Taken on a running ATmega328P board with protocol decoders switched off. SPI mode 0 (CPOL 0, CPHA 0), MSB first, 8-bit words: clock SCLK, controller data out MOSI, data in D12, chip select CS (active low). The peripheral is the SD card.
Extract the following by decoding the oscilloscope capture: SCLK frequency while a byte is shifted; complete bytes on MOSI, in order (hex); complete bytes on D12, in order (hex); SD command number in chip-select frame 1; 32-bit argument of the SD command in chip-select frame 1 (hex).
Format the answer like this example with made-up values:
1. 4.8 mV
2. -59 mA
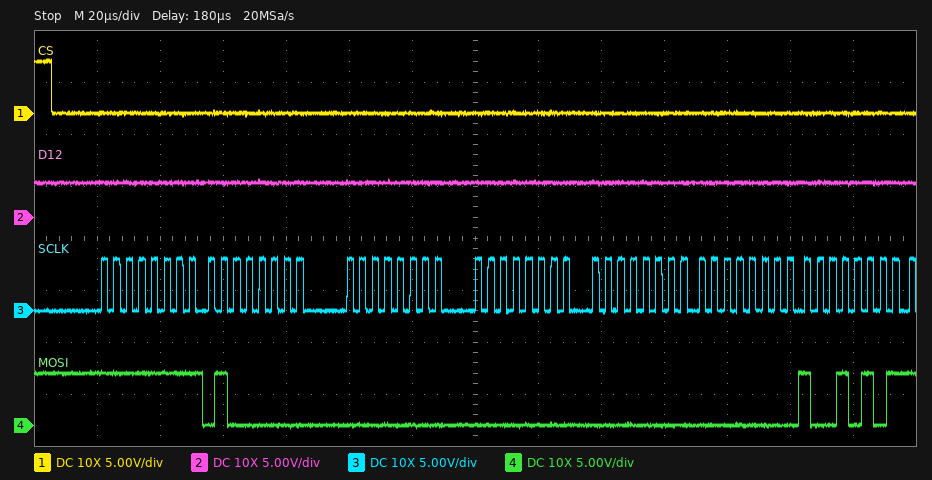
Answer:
1. 250 kHz
2. FF 40 00 00 00 00 95
3. FF FF FF FF FF FF FF
4. CMD0
5. 0x00000000
